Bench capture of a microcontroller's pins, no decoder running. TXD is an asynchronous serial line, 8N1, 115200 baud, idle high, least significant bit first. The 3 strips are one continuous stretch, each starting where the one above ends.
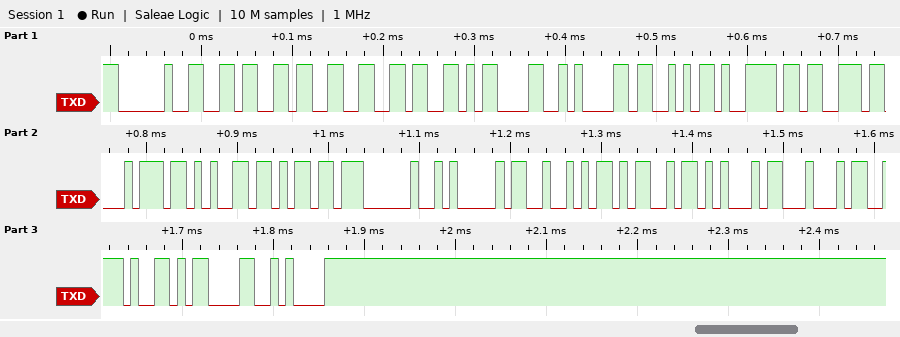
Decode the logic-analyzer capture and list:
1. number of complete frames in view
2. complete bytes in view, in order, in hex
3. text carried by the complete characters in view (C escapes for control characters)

21
20 36 33 36 0D 0A 53 79 73 74 65 6D 20 41 52 4D 45 44 2E 0D 0A
" 636\r\nSystem ARMED.\r\n"
